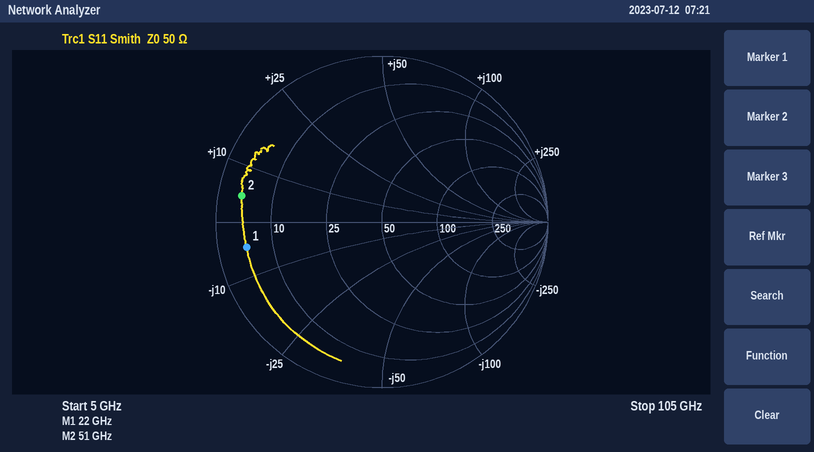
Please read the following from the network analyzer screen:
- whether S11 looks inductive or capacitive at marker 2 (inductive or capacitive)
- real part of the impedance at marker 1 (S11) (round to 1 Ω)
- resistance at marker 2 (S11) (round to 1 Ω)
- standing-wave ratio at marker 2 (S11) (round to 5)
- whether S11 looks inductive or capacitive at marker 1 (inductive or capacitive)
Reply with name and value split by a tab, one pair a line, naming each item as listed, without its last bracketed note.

whether S11 looks inductive or capacitive at marker 2	inductive
real part of the impedance at marker 1 (S11)	5 Ω
resistance at marker 2 (S11)	4 Ω
standing-wave ratio at marker 2 (S11)	15
whether S11 looks inductive or capacitive at marker 1	capacitive
